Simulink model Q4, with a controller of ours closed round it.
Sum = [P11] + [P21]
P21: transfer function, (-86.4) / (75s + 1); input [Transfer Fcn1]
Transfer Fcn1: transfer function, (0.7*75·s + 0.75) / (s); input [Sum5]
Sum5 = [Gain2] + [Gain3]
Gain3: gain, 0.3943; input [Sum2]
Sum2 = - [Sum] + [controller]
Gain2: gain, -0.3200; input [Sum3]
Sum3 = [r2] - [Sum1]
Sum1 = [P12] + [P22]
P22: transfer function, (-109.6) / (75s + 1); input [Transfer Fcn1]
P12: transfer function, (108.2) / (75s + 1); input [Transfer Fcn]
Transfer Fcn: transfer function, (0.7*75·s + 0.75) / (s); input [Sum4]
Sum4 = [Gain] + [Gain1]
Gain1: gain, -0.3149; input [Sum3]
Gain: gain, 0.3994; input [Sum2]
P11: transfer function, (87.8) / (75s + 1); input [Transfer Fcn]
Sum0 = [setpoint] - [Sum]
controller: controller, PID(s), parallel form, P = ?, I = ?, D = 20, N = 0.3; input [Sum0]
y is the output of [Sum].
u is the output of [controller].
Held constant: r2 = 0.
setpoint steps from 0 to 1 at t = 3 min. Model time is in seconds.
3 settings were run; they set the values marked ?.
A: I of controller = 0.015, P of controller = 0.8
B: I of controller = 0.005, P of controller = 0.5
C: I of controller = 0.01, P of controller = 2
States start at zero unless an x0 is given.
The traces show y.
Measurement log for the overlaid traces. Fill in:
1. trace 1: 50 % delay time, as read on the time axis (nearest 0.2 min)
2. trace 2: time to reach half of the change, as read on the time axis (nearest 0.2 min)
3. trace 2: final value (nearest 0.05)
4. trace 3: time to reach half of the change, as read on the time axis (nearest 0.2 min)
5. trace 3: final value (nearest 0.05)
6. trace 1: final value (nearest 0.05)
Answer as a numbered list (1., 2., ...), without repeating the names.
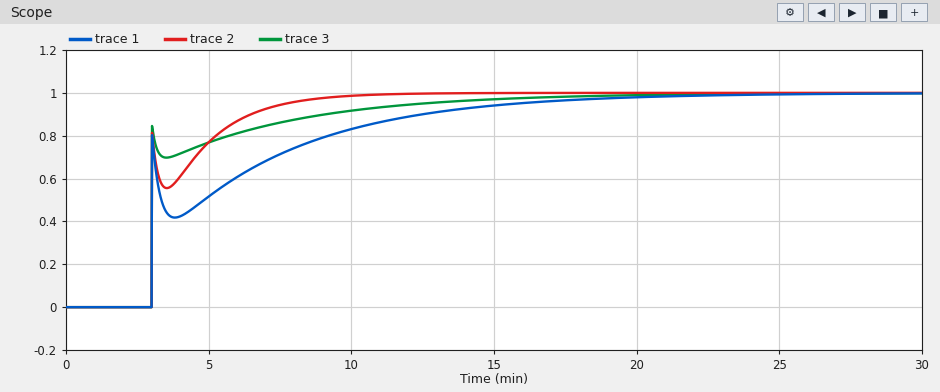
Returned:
1. 3.0 min
2. 3.0 min
3. 1.00
4. 3.0 min
5. 1.00
6. 1.00
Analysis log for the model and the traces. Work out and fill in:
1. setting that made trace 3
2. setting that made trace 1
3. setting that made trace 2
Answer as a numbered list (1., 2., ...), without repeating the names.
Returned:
1. C
2. B
3. A
